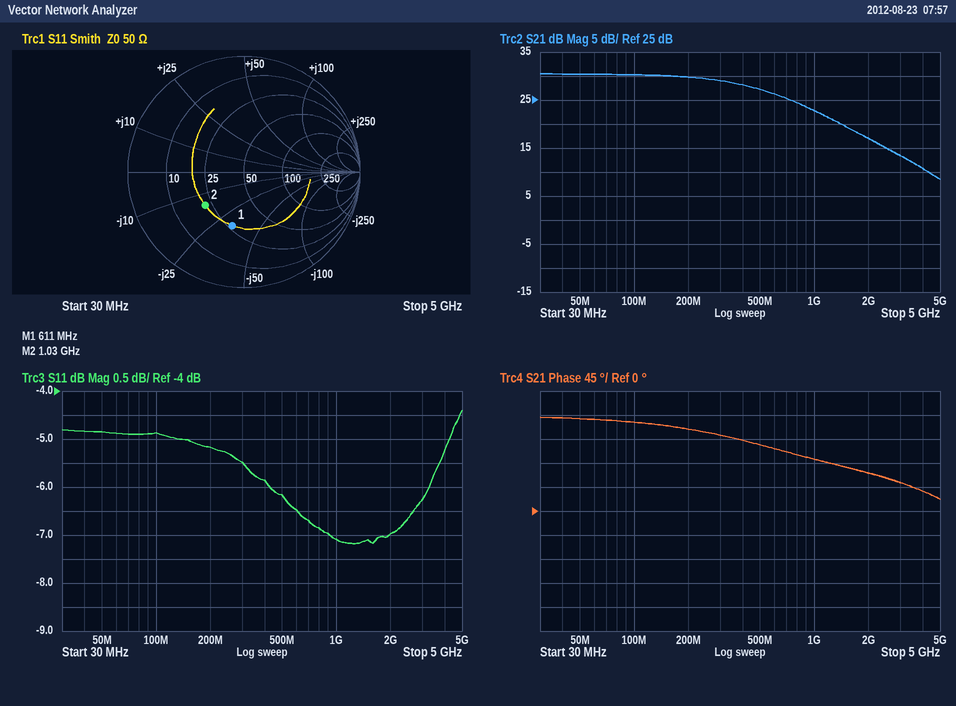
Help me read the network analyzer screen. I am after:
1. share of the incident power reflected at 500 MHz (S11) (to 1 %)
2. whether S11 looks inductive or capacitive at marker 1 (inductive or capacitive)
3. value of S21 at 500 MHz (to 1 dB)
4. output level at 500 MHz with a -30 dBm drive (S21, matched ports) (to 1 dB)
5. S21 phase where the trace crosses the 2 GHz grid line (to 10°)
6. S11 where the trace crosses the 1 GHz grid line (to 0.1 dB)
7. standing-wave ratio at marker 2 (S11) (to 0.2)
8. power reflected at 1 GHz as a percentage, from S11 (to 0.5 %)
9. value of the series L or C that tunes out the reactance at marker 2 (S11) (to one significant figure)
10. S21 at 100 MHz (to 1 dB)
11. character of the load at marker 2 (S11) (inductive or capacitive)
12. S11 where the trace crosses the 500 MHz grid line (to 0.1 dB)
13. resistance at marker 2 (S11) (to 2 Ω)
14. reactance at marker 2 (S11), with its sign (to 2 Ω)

24 %
capacitive
27 dB
-3 dBm
70°
-7.1 dB
2.6
19.5 %
2 nH
30 dB
capacitive
-6.2 dB
22 Ω
-16 Ω
